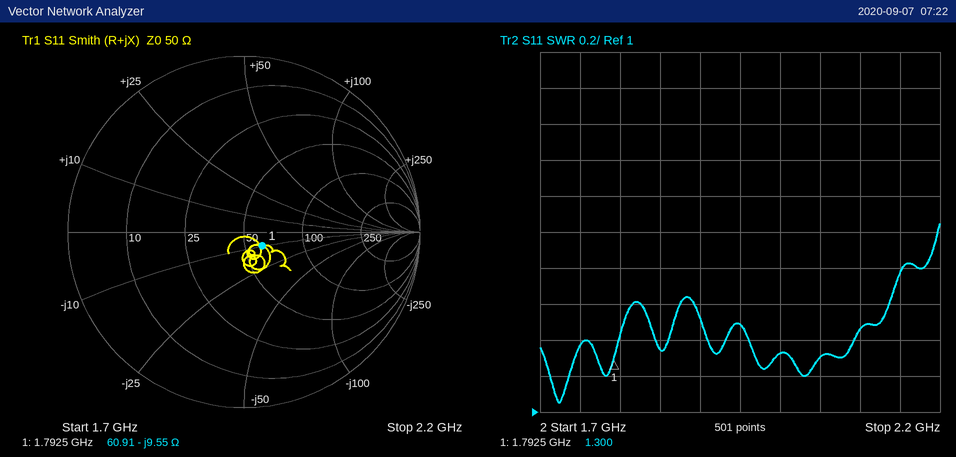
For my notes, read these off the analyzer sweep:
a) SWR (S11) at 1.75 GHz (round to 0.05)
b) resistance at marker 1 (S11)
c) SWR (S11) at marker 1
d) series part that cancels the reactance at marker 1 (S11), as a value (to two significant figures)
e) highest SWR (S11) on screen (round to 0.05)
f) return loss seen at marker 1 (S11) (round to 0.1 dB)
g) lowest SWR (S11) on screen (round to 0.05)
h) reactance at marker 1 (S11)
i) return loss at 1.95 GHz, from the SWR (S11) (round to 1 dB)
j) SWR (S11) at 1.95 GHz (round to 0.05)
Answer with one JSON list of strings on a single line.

["1.35", "60.91 Ω", "1.300", "850 pH", "2.05", "17.7 dB", "1.05", "-9.55 Ω", "14 dB", "1.50"]
